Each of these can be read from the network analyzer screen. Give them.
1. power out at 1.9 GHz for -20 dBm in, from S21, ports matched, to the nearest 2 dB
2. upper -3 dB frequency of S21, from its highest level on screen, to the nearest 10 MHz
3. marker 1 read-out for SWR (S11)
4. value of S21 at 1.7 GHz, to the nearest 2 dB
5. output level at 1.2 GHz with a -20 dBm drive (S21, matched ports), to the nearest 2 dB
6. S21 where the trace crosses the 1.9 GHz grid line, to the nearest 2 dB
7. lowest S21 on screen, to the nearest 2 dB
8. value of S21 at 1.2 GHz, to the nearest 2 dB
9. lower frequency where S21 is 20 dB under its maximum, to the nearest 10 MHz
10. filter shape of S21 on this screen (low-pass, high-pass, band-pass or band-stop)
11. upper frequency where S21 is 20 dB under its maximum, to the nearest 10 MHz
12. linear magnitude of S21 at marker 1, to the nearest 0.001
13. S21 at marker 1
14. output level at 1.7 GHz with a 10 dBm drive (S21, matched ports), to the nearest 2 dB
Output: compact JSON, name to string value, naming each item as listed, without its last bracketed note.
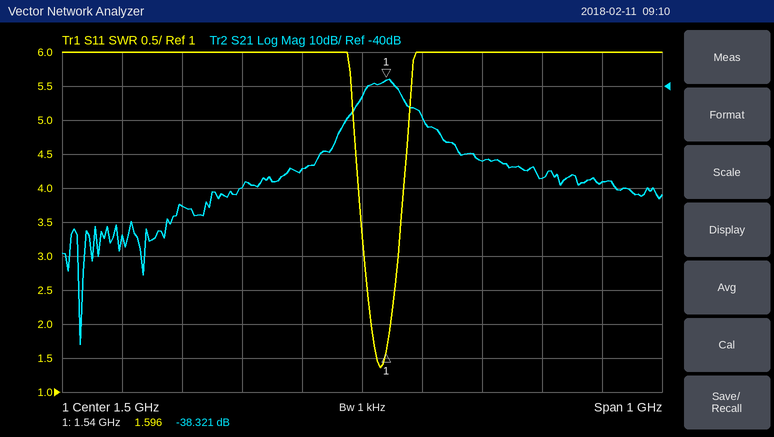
{"power out at 1.9 GHz for -20 dBm in, from S21, ports matched, to the nearest 2 dB": "-88 dBm", "upper -3 dB frequency of S21, from its highest level on screen, to the nearest 10 MHz": "1.56 GHz", "marker 1 read-out for SWR": "1.596", "value of S21 at 1.7 GHz, to the nearest 2 dB": "-62 dB", "output level at 1.2 GHz with a -20 dBm drive (S21, matched ports), to the nearest 2 dB": "-96 dBm", "S21 where the trace crosses the 1.9 GHz grid line, to the nearest 2 dB": "-68 dB", "lowest S21 on screen, to the nearest 2 dB": "-116 dB", "value of S21 at 1.2 GHz, to the nearest 2 dB": "-76 dB", "lower frequency where S21 is 20 dB under its maximum, to the nearest 10 MHz": "1.45 GHz", "filter shape of S21 on this screen": "band-pass", "upper frequency where S21 is 20 dB under its maximum, to the nearest 10 MHz": "1.66 GHz", "linear magnitude of S21 at marker 1, to the nearest 0.001": "0.012", "S21 at marker 1": "-38.321 dB", "output level at 1.7 GHz with a 10 dBm drive (S21, matched ports), to the nearest 2 dB": "-52 dBm"}
